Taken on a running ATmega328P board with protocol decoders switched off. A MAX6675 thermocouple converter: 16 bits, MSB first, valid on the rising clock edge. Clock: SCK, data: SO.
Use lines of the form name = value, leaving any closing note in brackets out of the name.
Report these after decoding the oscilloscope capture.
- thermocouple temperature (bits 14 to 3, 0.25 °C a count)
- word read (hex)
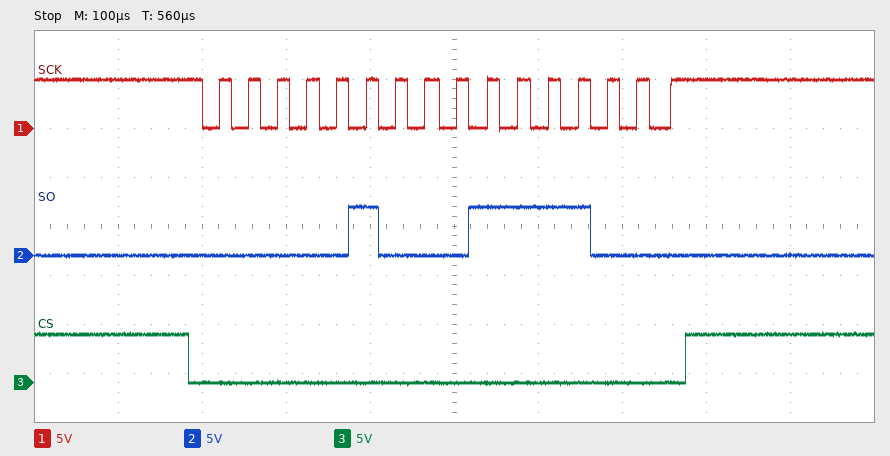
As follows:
thermocouple temperature = 35.75 °C
word read = 0x0478
